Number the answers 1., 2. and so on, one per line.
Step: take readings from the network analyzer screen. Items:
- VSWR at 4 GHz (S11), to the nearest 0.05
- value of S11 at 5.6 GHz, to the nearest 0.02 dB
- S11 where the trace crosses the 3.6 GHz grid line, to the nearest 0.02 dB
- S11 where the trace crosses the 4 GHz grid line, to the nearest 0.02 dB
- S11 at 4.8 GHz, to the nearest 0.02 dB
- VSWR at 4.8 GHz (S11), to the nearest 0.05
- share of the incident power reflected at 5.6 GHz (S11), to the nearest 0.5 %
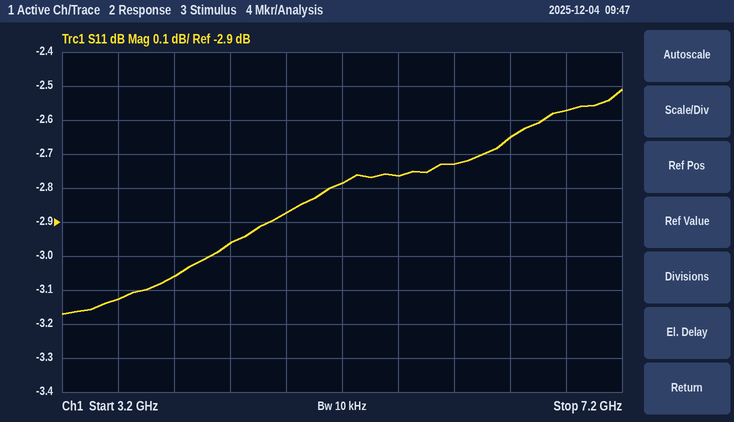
1. 5.75
2. -2.76 dB
3. -3.12 dB
4. -3.06 dB
5. -2.88 dB
6. 6.10
7. 53.0 %
